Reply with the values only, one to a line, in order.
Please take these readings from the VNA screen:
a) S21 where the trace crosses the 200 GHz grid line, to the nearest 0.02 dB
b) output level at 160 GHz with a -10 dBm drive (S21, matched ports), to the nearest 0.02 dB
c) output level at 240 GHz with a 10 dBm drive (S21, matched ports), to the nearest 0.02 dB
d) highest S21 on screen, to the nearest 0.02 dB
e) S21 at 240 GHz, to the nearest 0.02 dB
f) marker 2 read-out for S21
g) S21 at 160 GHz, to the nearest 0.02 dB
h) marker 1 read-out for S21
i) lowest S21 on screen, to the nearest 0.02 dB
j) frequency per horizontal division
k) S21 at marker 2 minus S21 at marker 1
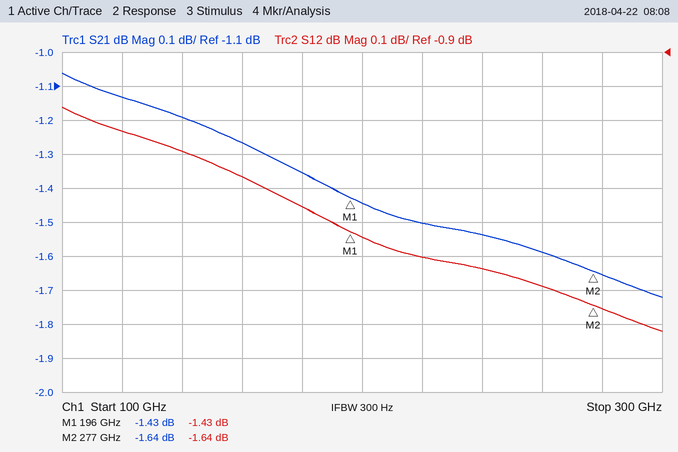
-1.44 dB
-11.26 dBm
8.46 dBm
-1.06 dB
-1.54 dB
-1.64 dB
-1.26 dB
-1.43 dB
-1.72 dB
20 GHz
-0.21 dB
